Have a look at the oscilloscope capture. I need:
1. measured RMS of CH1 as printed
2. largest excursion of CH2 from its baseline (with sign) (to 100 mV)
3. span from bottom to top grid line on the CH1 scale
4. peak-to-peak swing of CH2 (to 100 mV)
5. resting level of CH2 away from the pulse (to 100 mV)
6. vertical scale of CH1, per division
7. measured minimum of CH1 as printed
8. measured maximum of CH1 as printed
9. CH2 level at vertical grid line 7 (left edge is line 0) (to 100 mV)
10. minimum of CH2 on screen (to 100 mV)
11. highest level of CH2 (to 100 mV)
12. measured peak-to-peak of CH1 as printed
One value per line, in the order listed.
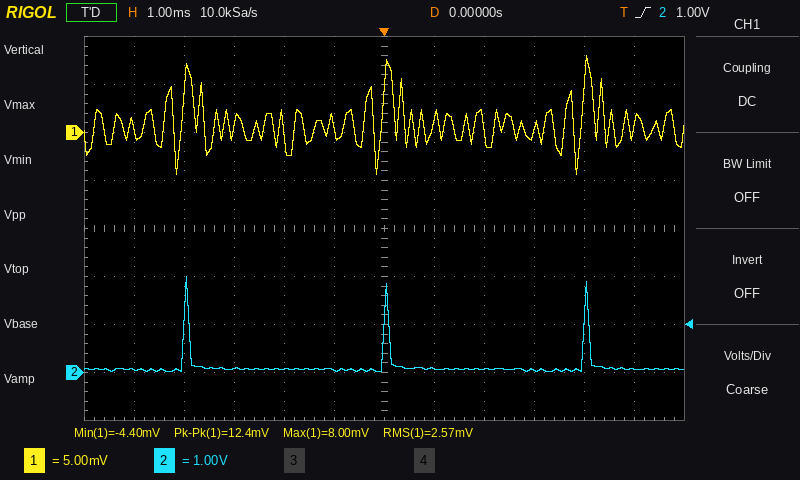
2.57 mV
+1.9 V
40 mV
2.0 V
100 mV
5 mV
-4.40 mV
8.00 mV
100 mV
0.0 V
2.0 V
12.4 mV
